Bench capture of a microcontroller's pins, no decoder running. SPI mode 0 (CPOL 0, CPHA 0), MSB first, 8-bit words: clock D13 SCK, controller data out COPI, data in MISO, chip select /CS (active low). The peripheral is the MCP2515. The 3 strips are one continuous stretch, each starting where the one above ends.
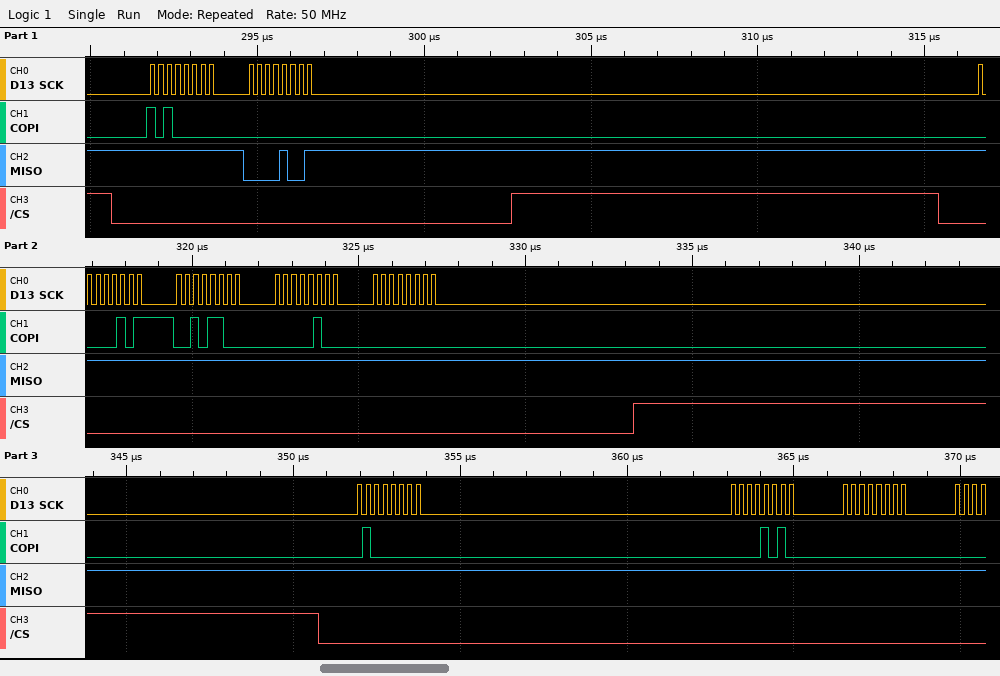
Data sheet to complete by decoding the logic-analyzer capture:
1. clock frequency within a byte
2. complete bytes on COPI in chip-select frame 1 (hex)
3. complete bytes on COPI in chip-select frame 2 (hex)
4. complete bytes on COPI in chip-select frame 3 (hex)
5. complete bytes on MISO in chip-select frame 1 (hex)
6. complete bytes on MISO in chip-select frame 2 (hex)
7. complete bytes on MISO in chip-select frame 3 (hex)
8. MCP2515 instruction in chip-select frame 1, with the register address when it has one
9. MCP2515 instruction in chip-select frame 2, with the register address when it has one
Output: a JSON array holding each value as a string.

["4 MHz", "0xA0 0x00", "0x05 0x2C 0x04 0x00", "0x40 0x0A 0x00", "0xFF 0x09", "0xFF 0xFF 0xFF 0xFF", "0xFF 0xFF 0xFF", "READ STATUS", "BIT MODIFY 0x2C"]
